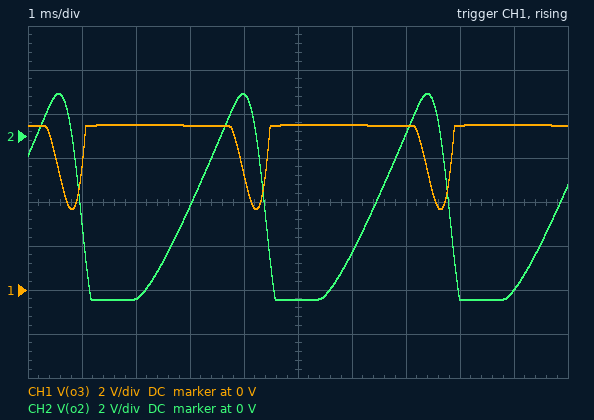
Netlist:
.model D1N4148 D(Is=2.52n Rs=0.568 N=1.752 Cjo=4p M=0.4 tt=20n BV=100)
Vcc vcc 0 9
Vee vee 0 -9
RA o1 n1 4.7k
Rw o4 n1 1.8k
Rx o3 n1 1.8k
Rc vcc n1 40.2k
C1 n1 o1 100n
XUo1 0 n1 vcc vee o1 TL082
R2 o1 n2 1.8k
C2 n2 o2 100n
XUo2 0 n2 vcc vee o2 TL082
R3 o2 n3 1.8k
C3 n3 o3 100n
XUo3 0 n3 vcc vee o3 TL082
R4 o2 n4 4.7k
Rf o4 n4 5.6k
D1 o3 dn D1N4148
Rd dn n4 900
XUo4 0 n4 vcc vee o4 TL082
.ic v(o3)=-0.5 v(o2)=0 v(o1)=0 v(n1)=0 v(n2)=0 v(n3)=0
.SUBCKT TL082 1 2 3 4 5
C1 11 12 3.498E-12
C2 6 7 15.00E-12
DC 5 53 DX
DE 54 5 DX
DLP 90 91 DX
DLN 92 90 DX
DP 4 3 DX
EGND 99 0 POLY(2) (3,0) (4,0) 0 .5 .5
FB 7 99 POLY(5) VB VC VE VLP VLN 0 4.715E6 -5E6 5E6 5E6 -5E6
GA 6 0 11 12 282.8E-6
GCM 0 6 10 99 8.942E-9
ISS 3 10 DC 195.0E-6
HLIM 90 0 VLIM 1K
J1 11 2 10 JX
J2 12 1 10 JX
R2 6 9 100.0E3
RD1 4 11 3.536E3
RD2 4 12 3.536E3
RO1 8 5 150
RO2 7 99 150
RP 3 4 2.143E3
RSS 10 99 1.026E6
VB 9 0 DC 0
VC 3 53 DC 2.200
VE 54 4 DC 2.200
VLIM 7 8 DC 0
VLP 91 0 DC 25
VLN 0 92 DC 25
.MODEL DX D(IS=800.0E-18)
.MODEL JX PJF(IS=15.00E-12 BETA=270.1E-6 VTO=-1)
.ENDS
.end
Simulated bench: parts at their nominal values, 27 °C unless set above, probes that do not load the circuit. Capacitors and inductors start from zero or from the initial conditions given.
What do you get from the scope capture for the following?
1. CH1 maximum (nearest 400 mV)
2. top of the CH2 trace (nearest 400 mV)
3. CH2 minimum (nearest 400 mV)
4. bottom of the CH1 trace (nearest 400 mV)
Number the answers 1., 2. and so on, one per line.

1. 7.6 V
2. 2.0 V
3. -7.6 V
4. 3.6 V
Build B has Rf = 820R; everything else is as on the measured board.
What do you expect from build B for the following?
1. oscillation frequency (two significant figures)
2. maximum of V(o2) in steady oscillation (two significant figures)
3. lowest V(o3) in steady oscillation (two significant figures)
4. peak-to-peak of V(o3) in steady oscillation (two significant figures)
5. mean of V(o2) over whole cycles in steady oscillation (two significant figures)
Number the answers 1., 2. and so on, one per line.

1. 510 Hz
2. 7.5 V
3. -7.5 V
4. 15 V
5. -1.3 V
